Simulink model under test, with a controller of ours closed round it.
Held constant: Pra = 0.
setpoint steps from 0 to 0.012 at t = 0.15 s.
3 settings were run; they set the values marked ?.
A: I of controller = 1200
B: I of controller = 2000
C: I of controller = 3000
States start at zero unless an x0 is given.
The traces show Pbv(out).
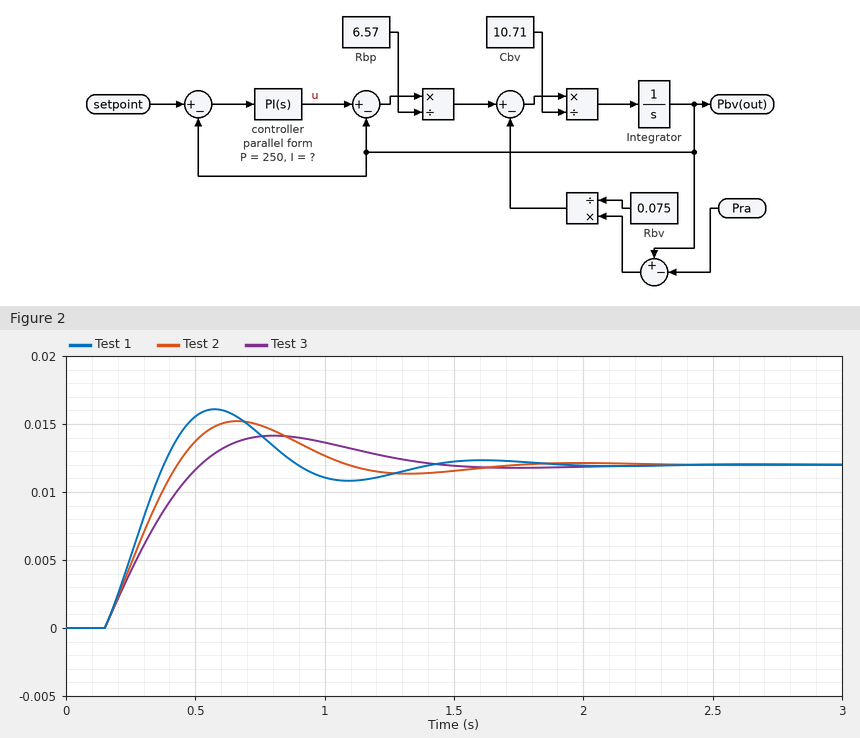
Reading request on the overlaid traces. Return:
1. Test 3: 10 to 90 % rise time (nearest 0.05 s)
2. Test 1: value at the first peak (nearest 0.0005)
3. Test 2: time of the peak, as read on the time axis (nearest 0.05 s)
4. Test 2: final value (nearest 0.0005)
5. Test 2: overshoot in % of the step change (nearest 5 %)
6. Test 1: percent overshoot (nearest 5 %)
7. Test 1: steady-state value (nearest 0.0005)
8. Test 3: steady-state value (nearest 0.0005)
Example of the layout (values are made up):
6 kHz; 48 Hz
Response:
0.30 s; 0.0160; 0.65 s; 0.0120; 25 %; 35 %; 0.0120; 0.0120
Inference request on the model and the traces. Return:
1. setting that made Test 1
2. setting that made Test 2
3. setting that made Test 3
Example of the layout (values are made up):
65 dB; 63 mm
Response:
C; B; A
